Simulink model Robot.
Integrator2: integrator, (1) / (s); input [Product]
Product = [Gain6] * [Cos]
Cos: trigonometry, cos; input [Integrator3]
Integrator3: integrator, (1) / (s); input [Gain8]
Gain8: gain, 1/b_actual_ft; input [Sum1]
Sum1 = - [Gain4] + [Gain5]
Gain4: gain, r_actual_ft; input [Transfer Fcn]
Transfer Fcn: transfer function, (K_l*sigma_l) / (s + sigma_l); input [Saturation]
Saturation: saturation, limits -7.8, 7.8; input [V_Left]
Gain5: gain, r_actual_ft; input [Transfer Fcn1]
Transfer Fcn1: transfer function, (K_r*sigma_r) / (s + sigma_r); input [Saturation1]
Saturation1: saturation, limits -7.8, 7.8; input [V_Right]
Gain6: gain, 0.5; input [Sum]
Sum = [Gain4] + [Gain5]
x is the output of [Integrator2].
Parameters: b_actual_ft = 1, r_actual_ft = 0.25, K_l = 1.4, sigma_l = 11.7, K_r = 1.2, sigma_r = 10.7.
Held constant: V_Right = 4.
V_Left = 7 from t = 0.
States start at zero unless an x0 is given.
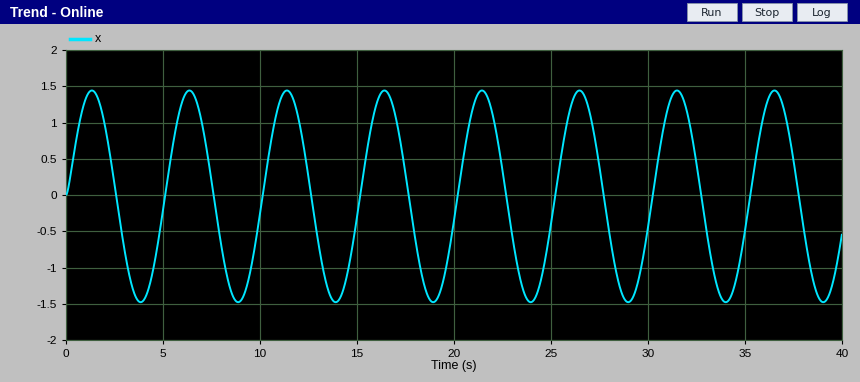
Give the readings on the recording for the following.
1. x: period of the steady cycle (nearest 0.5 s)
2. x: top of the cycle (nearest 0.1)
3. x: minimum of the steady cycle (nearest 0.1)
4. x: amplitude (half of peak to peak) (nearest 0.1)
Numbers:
5.0 s
1.4
-1.5
1.5
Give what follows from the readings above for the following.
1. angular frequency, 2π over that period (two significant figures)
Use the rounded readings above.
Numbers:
1.3 rad/s
